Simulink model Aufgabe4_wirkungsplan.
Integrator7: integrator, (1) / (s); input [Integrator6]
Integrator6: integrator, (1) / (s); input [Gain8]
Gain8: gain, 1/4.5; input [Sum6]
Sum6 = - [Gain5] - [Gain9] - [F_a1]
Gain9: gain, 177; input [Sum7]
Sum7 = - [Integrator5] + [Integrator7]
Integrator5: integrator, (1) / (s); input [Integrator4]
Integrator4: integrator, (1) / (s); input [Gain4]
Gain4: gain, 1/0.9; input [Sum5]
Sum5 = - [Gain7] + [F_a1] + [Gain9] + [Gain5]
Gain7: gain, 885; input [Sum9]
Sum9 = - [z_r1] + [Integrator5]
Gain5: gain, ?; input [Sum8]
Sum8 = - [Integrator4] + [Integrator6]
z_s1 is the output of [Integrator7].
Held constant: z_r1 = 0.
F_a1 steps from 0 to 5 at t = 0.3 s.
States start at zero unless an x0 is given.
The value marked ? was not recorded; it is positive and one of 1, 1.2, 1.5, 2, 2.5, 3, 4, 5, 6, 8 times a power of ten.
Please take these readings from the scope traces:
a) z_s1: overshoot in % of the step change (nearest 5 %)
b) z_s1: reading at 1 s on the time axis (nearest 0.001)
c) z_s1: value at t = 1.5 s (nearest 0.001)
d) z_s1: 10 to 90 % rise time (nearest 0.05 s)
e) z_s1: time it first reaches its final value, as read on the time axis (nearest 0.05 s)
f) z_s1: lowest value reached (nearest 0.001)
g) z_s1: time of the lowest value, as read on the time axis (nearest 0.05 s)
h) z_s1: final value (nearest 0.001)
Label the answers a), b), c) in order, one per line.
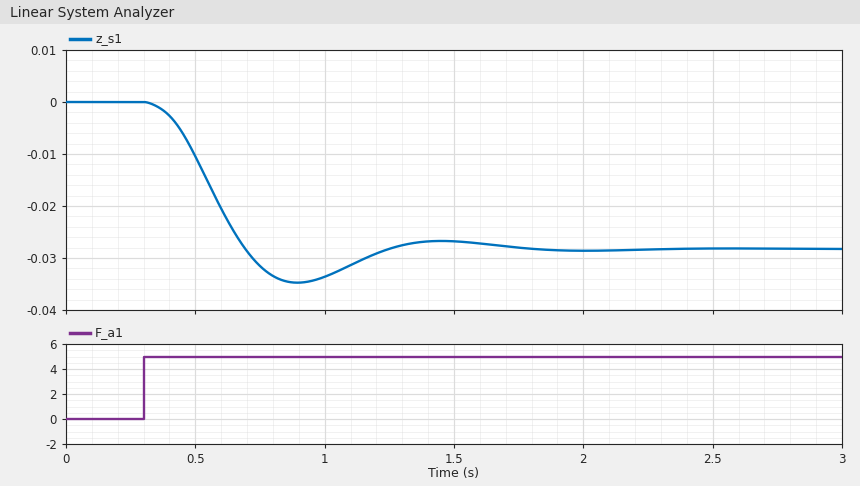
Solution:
a) 25 %
b) -0.034
c) -0.027
d) 0.25 s
e) 0.70 s
f) -0.035
g) 0.90 s
h) -0.028
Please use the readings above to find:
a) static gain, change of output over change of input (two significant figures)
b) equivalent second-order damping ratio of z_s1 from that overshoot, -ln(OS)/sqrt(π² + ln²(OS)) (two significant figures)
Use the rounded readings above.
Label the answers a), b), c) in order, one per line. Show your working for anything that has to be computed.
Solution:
a) (-0.028 - 0) / (5 - 0) = -0.0056
b) ln(0.25) = -1.386; 1.386 / sqrt(9.870 + 1.922) = 0.40
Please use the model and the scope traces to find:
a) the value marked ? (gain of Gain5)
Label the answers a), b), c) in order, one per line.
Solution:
a) 30
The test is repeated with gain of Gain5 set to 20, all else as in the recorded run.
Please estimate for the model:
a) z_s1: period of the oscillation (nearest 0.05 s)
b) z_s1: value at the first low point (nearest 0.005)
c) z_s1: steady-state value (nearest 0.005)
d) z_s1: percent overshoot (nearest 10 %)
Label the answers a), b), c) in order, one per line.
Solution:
a) 1.10 s
b) -0.040
c) -0.030
d) 40 %
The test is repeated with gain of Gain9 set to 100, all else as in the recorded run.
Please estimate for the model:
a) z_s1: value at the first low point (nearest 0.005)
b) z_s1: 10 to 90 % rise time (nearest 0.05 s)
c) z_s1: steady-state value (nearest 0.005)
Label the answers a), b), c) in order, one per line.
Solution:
a) -0.055
b) 0.40 s
c) -0.050
